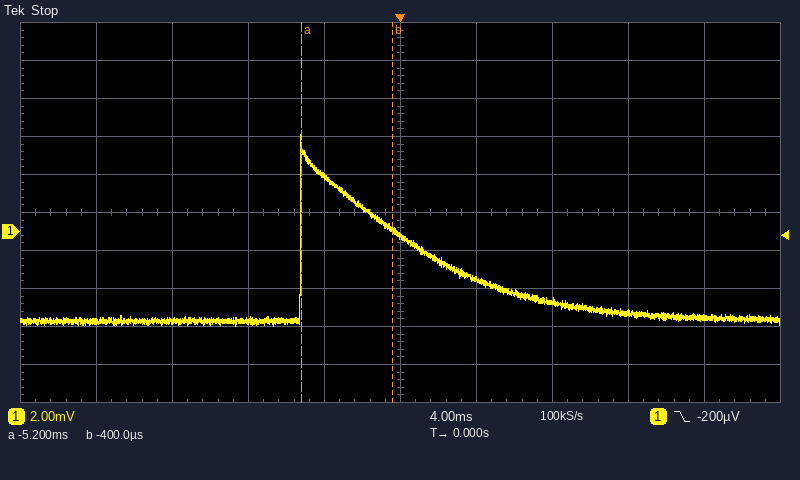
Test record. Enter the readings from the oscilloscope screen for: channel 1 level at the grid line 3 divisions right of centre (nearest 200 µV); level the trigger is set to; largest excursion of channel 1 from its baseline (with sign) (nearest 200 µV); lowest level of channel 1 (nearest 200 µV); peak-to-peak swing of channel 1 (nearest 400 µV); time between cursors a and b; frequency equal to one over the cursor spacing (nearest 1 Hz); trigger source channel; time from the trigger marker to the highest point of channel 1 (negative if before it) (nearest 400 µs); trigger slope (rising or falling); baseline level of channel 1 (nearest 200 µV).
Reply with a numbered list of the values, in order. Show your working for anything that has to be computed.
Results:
1. -4.2 mV
2. -200 µV
3. +9.8 mV
4. -5.0 mV
5. 10.0 mV
6. -400 µs − (-5.2 ms) = 4.8 ms
7. 1 / 4.8 ms ≈ 208 Hz
8. channel 1
9. -5.2 ms
10. falling
11. -4.6 mV
